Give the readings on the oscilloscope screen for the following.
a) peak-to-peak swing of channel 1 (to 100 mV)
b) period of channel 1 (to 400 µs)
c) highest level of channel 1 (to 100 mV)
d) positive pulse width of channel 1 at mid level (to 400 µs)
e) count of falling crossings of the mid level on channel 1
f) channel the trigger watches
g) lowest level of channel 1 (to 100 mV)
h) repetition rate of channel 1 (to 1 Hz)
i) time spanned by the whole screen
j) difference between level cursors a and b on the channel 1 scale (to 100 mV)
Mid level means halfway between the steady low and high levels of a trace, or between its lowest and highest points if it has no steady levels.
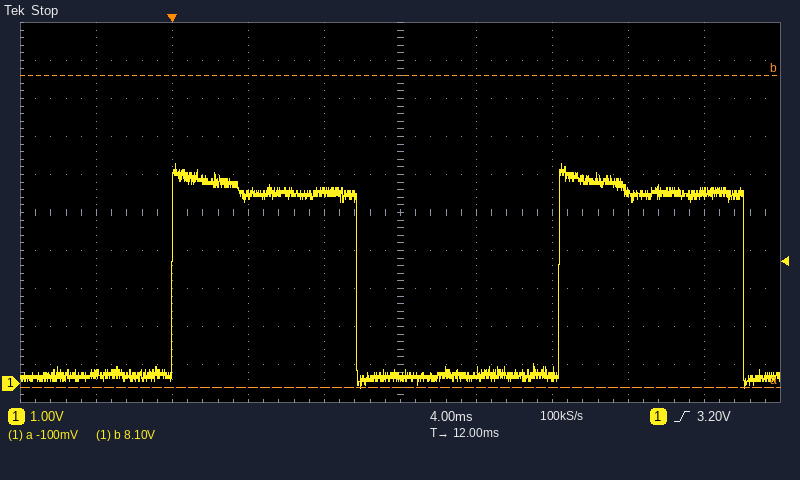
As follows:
5.9 V
20.4 ms
5.8 V
9.6 ms
2
channel 1
-100 mV
49 Hz
40 ms
8.2 V
